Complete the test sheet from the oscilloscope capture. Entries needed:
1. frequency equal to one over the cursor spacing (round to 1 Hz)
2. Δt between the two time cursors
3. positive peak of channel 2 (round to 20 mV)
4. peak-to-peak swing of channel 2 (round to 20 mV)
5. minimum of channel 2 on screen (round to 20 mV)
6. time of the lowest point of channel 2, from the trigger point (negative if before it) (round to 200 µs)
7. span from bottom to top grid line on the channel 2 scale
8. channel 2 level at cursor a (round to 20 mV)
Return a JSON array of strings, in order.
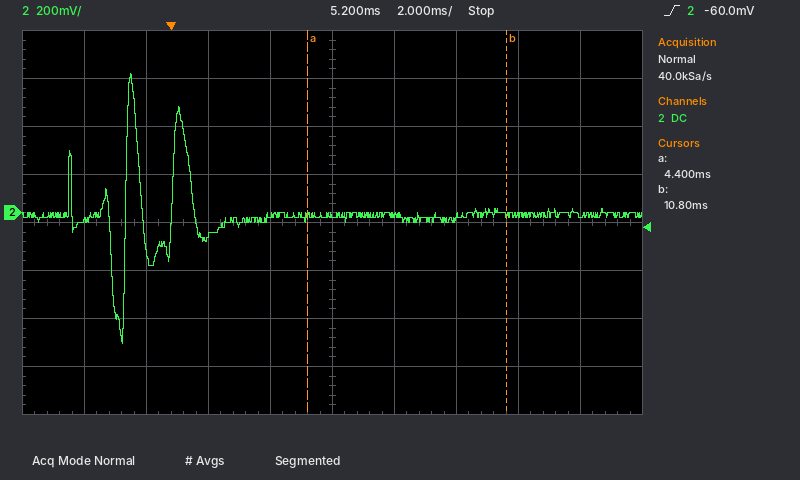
["156 Hz", "6.4 ms", "580 mV", "1.12 V", "-540 mV", "-1.6 ms", "1.6 V", "-20 mV"]
